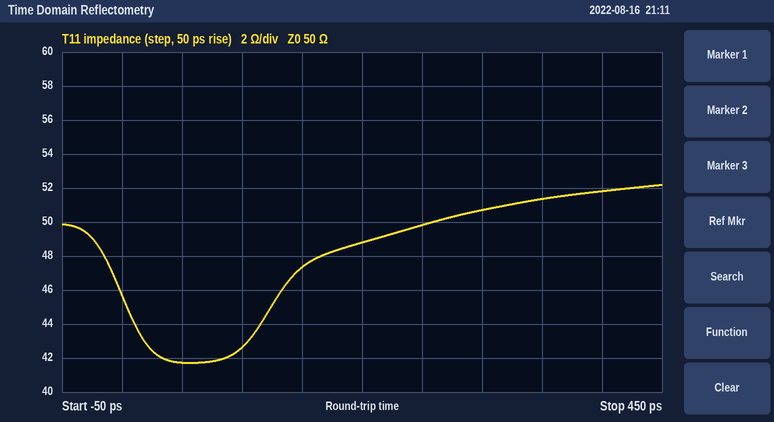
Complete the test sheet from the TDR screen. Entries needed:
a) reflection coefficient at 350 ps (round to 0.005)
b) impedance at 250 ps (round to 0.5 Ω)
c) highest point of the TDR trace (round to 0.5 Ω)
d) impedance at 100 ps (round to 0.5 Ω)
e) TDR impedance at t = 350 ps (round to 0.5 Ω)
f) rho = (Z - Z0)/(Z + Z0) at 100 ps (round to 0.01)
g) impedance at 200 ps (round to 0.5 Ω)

+0.015
50.0 Ω
52.0 Ω
42.5 Ω
51.5 Ω
-0.08
49.0 Ω
